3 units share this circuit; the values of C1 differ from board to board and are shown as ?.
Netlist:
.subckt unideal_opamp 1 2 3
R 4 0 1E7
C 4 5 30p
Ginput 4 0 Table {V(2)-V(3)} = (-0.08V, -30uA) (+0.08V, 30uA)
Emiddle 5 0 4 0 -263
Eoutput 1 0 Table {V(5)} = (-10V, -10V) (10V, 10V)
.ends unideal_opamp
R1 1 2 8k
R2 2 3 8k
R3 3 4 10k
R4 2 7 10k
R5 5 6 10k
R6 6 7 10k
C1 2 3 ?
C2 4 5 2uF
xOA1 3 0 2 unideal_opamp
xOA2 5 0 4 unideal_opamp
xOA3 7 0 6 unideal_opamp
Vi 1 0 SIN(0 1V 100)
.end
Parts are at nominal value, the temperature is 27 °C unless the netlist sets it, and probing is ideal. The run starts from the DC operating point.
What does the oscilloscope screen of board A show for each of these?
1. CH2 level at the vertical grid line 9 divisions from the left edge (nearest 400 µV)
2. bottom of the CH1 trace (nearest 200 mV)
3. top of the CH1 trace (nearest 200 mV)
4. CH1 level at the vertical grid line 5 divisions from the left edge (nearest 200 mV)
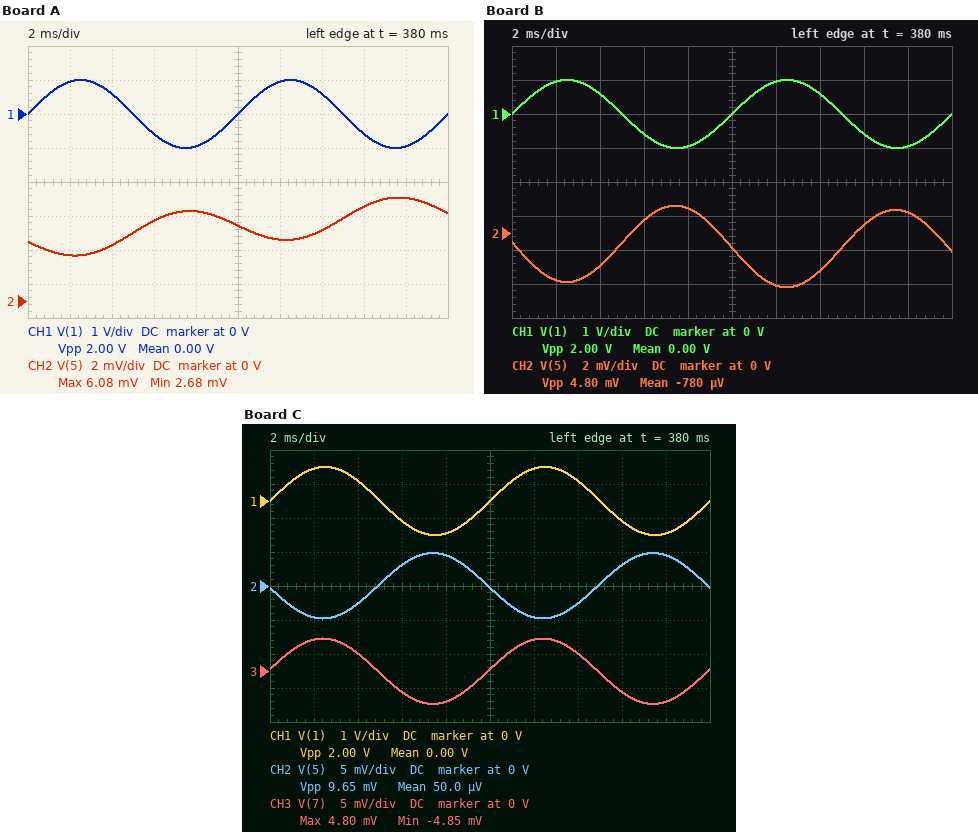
6.0 mV
-1.0 V
1.0 V
0 V
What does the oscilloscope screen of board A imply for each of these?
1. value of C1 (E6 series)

15 µF
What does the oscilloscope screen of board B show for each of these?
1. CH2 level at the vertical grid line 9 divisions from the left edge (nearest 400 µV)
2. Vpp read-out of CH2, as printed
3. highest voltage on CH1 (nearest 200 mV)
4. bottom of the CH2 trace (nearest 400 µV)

1.2 mV
4.80 mV
1.0 V
-3.2 mV
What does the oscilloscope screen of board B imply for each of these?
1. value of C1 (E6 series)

6.8 µF
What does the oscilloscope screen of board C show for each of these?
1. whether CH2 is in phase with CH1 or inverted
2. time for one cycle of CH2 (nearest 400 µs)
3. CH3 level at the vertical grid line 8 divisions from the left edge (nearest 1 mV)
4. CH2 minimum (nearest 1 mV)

inverted
10.0 ms
-3 mV
-5 mV
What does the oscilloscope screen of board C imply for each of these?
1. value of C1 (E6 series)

3.3 µF
